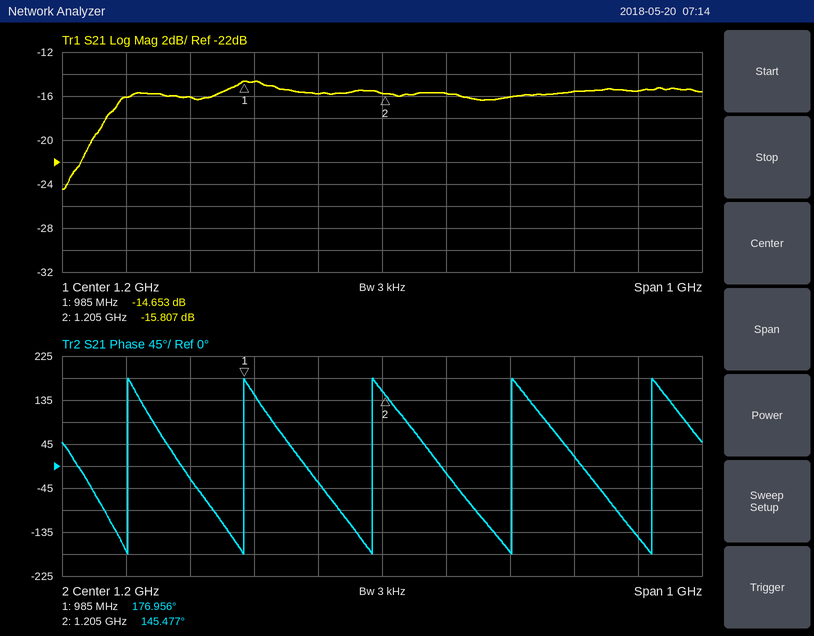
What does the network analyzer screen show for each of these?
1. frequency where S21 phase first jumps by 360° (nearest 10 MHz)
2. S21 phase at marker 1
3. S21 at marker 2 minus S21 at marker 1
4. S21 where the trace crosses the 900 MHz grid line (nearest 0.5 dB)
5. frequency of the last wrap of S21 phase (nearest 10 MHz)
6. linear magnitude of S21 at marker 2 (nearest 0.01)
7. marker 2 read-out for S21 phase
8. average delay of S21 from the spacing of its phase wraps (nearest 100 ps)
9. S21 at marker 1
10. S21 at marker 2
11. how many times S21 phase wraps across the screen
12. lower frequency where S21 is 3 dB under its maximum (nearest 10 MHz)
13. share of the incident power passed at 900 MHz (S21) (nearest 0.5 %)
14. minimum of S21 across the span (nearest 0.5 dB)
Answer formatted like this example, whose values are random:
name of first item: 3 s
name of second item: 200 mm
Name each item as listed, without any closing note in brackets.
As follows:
frequency where S21 phase first jumps by 360°: 800 MHz
S21 phase at marker 1: 176.956°
S21 at marker 2 minus S21 at marker 1: -1.154 dB
S21 where the trace crosses the 900 MHz grid line: -16.0 dB
frequency of the last wrap of S21 phase: 1.62 GHz
linear magnitude of S21 at marker 2: 0.16
marker 2 read-out for S21 phase: 145.477°
average delay of S21 from the spacing of its phase wraps: 4.9 ns
S21 at marker 1: -14.653 dB
S21 at marker 2: -15.807 dB
how many times S21 phase wraps across the screen: 5
lower frequency where S21 is 3 dB under its maximum: 770 MHz
share of the incident power passed at 900 MHz (S21): 2.5 %
minimum of S21 across the span: -24.5 dB
